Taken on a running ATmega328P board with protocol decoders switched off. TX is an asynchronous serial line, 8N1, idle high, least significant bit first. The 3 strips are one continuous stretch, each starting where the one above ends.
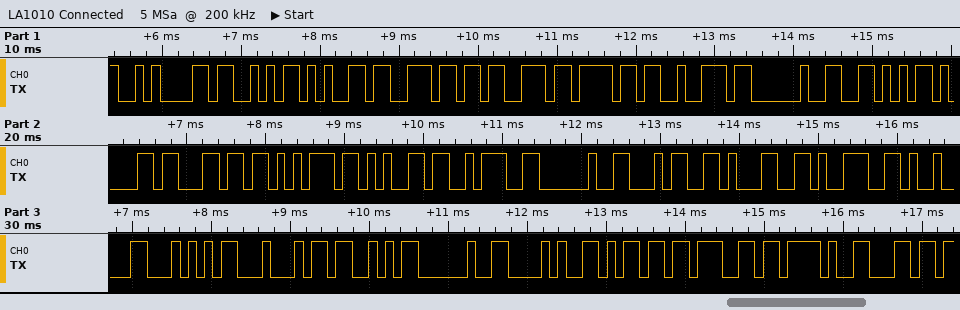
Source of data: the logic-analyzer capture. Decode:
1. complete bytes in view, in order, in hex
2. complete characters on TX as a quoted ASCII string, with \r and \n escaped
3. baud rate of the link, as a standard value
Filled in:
0A 53 65 6E 73 6F 72 20 56 61 6C 75 65 3A 20 34 31 39 09 54 44 53 20 28 6D 67 2F 6C
"\nSensor Value: 419\tTDS (mg/l"
9600 baud
